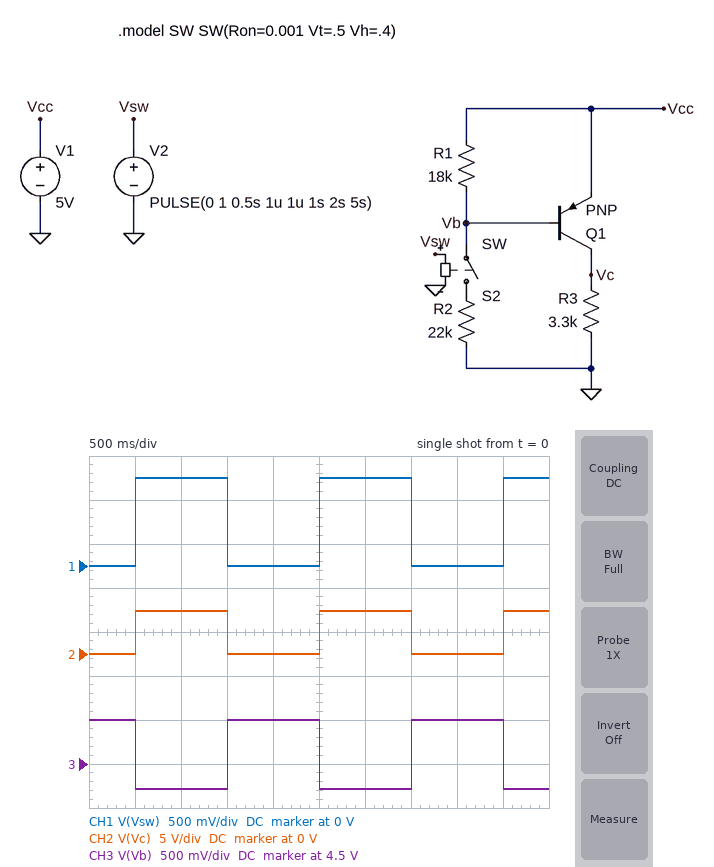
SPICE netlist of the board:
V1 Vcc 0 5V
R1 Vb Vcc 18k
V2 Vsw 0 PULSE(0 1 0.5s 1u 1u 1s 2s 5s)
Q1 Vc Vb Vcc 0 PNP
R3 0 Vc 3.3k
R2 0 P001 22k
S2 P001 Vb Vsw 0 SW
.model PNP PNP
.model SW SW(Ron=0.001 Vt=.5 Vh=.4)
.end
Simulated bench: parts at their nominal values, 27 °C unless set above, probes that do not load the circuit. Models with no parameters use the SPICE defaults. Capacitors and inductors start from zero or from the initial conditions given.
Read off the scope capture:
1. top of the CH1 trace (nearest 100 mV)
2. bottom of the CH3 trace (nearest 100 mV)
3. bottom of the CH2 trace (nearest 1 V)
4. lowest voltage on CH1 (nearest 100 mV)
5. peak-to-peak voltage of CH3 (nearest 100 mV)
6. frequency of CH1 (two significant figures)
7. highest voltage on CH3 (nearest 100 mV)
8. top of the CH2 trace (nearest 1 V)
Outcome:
1.0 V
4.2 V
0 V
0 V
800 mV
500 mHz
5.0 V
5 V
